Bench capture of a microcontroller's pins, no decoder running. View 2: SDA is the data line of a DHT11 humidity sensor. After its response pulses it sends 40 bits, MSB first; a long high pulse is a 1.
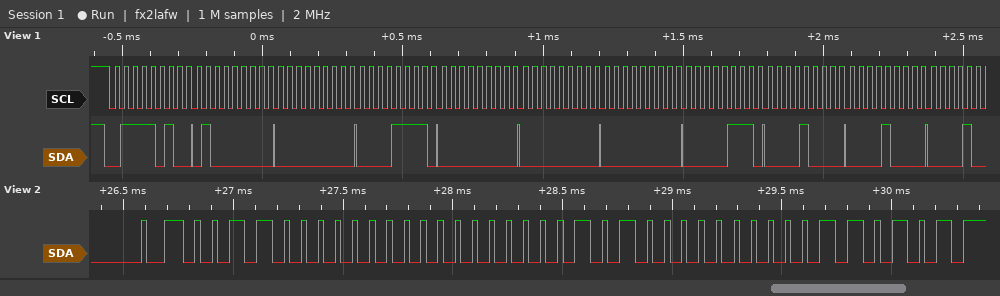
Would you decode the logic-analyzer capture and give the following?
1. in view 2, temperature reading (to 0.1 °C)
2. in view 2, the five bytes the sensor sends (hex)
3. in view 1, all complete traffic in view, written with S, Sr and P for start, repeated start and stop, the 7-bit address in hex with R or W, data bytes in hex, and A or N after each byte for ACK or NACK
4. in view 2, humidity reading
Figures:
5.0 °C
30 00 05 00 35
S 3DW A 40 A 00 A 0F A 00 A 00 A 00 A 07 A 08 A 08 A
48 %
